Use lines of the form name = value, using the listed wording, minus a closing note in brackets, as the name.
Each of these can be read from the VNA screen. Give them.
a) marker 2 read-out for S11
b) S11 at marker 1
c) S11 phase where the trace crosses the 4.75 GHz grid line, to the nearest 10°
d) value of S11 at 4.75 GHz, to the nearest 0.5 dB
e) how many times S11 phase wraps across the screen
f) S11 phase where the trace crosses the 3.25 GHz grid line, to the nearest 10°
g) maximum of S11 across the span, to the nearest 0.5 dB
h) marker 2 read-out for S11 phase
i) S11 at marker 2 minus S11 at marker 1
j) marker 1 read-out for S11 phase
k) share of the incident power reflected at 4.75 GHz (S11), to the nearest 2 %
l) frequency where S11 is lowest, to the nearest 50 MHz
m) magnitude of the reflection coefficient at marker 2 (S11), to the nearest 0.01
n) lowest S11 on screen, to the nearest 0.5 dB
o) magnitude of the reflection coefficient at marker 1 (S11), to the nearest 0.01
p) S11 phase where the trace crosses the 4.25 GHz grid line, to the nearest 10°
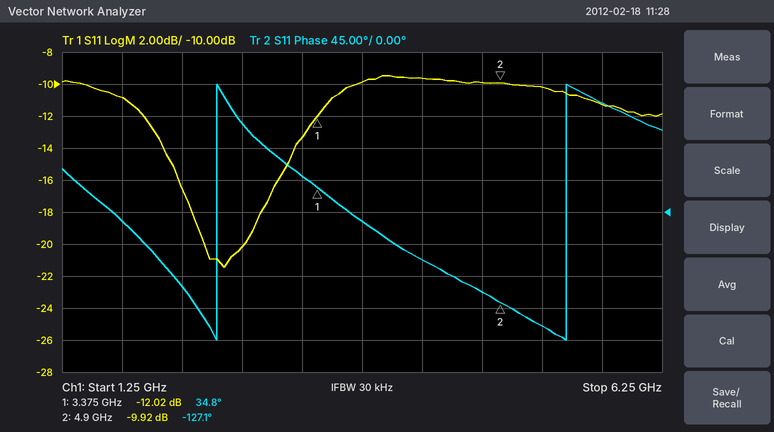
marker 2 read-out for S11 = -9.92 dB
S11 at marker 1 = -12.02 dB
S11 phase where the trace crosses the 4.75 GHz grid line, to the nearest 10° = -110°
value of S11 at 4.75 GHz, to the nearest 0.5 dB = -10.0 dB
how many times S11 phase wraps across the screen = 2
S11 phase where the trace crosses the 3.25 GHz grid line, to the nearest 10° = 50°
maximum of S11 across the span, to the nearest 0.5 dB = -9.5 dB
marker 2 read-out for S11 phase = -127.1°
S11 at marker 2 minus S11 at marker 1 = 2.10 dB
marker 1 read-out for S11 phase = 34.8°
share of the incident power reflected at 4.75 GHz (S11), to the nearest 2 % = 10 %
frequency where S11 is lowest, to the nearest 50 MHz = 2.60 GHz
magnitude of the reflection coefficient at marker 2 (S11), to the nearest 0.01 = 0.32
lowest S11 on screen, to the nearest 0.5 dB = -21.5 dB
magnitude of the reflection coefficient at marker 1 (S11), to the nearest 0.01 = 0.25
S11 phase where the trace crosses the 4.25 GHz grid line, to the nearest 10° = -70°
